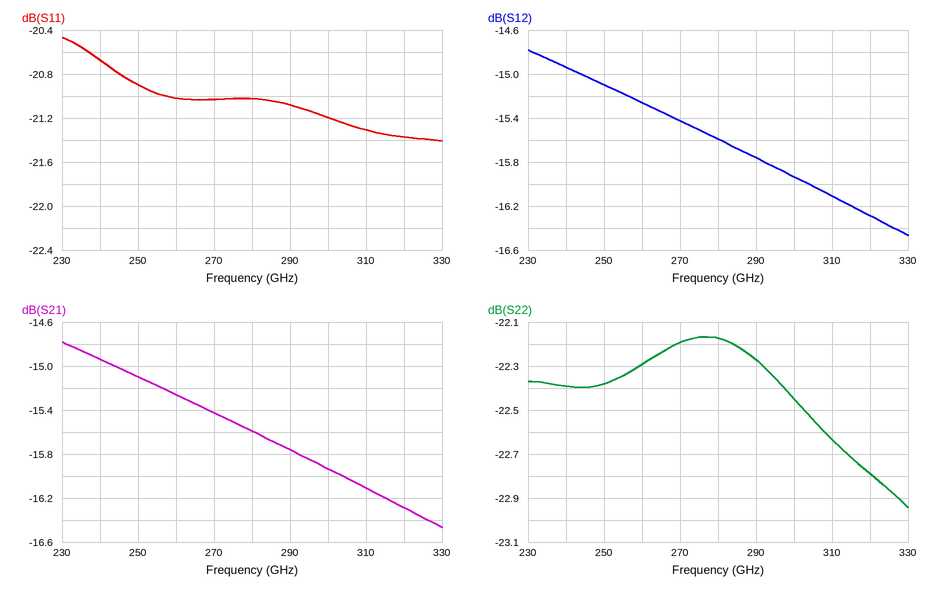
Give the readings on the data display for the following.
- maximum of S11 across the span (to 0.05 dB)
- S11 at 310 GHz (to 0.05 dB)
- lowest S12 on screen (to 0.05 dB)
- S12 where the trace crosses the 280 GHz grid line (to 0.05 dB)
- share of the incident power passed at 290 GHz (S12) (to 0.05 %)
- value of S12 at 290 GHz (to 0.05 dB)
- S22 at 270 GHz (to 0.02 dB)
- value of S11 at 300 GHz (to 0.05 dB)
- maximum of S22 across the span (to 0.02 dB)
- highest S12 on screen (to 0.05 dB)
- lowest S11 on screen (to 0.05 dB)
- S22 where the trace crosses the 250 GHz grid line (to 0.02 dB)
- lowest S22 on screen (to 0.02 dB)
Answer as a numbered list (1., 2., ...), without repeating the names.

1. -20.45 dB
2. -21.30 dB
3. -16.45 dB
4. -15.60 dB
5. 2.65 %
6. -15.75 dB
7. -22.20 dB
8. -21.20 dB
9. -22.16 dB
10. -14.80 dB
11. -21.40 dB
12. -22.38 dB
13. -22.94 dB
